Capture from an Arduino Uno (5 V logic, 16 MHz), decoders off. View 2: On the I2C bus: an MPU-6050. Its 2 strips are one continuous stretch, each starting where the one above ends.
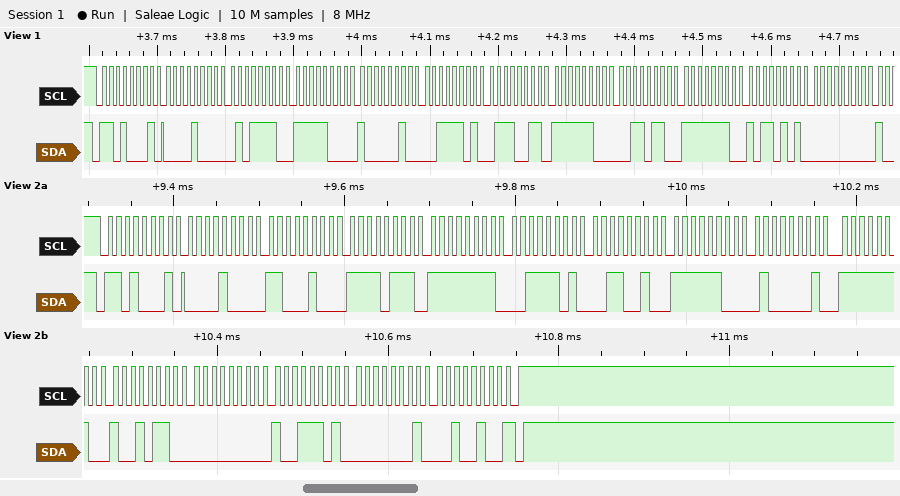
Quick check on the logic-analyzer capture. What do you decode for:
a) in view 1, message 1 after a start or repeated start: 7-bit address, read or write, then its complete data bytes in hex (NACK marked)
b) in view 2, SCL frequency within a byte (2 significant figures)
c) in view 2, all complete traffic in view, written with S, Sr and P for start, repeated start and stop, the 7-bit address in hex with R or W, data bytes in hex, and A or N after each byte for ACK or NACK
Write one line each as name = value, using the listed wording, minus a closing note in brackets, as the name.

in view 1, message 1 after a start or repeated start: 7-bit address, read or write, then its complete data bytes in hex = 0x68 read: 08 5E F8 82 3D 73 FC 36 FE B5 00
in view 2, SCL frequency within a byte = 100 kHz
in view 2, all complete traffic in view, written with S, Sr and P for start, repeated start and stop, the 7-bit address in hex with R or W, data bytes in hex, and A or N after each byte for ACK or NACK = S 68R A 08 A C4 A F7 A FF A 3D A 32 A FC A 41 A FE A 96 A 00 A 9D A 01 A 24 N P
